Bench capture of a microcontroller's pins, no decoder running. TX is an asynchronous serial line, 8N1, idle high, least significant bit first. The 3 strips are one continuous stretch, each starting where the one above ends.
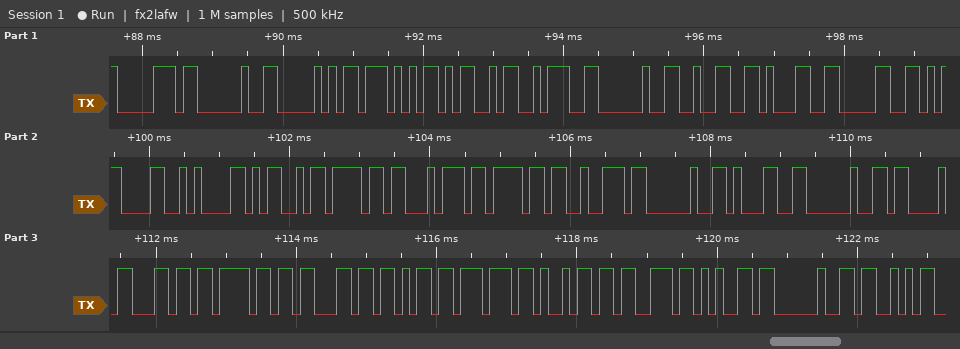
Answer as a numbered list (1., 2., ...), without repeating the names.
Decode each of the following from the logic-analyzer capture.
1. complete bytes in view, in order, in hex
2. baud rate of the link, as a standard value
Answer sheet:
1. 0x70 0x20 0x50 0x57 0x4D 0x3A 0x20 0x32 0x31 0x30 0x0D 0x0A 0x4D 0x6F 0x74 0x6F 0x72 0x20 0x31 0x20 0x43 0x6C 0x6F 0x63 0x6B 0x77 0x69 0x73 0x65 0x20 0x53
2. 9600 baud
